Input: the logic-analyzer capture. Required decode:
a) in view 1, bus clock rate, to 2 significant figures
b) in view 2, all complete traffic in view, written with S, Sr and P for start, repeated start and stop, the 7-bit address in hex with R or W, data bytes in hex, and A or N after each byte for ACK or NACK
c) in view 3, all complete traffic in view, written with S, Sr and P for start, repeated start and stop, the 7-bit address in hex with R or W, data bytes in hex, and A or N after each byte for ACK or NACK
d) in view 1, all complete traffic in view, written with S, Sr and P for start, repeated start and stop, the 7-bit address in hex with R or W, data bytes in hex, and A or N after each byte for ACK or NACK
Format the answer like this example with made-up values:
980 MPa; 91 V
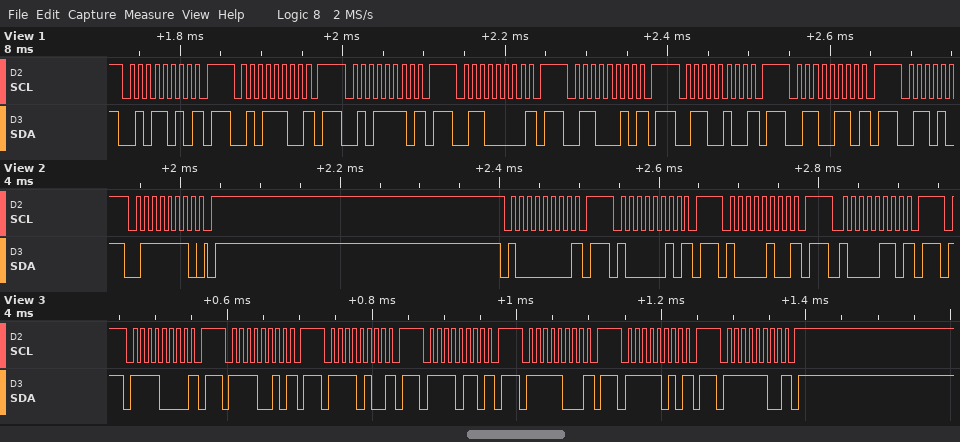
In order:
100 kHz; S 3FW A P S 40W N P S 41W N P S 42W N P S 43W N P; S 78W N P S 79W N P S 7AW N P S 7BW N P S 7CW N P S 7DW N P S 7EW N P; S 2DW N P S 2EW N P S 2FW N P S 30W N P S 31W N P S 32W N P S 33W N P
